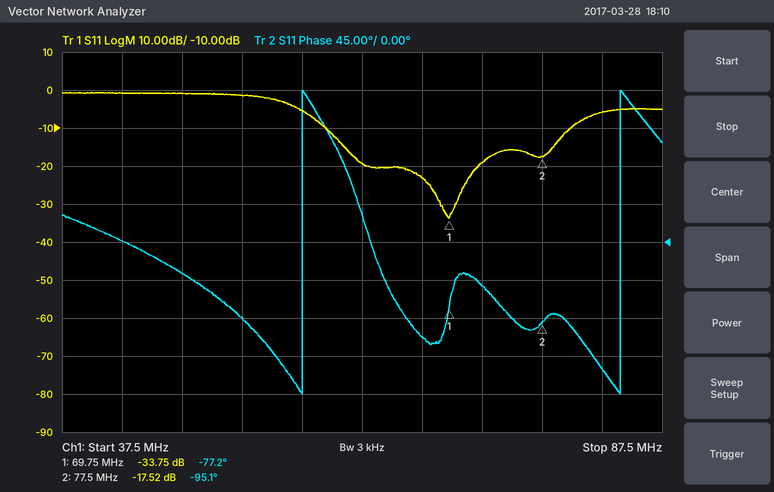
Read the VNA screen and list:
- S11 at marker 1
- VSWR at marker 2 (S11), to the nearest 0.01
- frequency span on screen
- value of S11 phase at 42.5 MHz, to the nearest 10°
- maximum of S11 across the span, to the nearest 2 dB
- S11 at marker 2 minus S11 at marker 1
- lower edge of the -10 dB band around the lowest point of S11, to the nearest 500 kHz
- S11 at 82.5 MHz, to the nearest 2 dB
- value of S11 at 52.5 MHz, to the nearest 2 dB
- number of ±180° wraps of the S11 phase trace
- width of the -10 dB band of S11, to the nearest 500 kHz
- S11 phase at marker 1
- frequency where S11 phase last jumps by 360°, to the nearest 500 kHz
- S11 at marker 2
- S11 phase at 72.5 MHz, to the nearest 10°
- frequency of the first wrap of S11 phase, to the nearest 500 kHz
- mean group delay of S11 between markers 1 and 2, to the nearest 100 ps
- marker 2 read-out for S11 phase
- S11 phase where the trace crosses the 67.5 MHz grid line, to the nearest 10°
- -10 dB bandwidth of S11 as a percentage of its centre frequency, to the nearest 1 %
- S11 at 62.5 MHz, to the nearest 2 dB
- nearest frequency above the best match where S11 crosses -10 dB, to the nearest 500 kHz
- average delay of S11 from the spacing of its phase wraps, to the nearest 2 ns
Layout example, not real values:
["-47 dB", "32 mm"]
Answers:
["-33.75 dB", "1.31", "50 MHz", "0°", "0 dB", "16.23 dB", "59.5 MHz", "-6 dB", "-2 dB", "2", "20.5 MHz", "-77.2°", "84.0 MHz", "-17.52 dB", "-50°", "57.5 MHz", "6.4 ns", "-95.1°", "-110°", "29 %", "-20 dB", "80.0 MHz", "38 ns"]
